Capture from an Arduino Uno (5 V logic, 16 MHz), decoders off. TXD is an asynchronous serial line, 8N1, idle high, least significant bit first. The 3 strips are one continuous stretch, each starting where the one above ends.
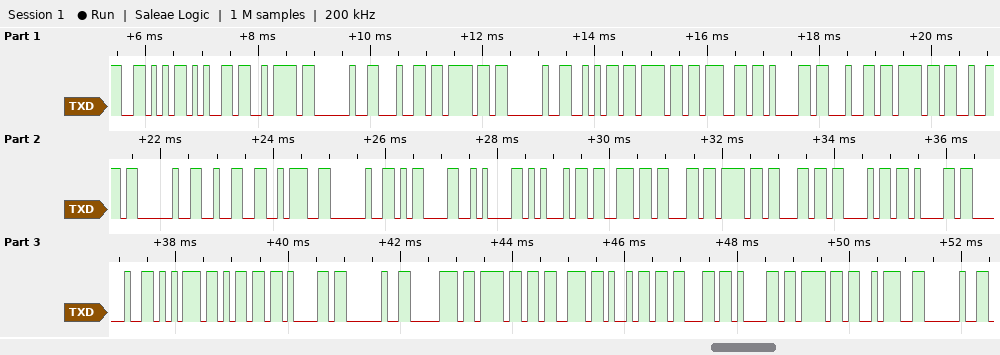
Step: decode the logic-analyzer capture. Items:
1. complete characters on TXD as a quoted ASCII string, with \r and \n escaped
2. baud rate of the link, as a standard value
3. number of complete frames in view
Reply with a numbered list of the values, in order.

1. "Vez do jogador 2: \r\nEscolha uma posicao: "
2. 9600 baud
3. 41
